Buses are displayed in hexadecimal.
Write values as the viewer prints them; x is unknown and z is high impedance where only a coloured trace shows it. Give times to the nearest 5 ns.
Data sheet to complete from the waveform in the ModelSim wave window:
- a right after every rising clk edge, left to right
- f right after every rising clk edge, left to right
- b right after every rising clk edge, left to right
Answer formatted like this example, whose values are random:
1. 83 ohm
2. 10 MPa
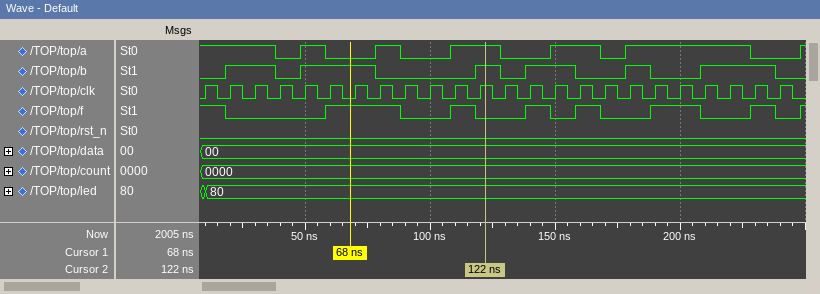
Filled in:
1. 1 1 1 0 1 0 0 1 0 0 1 1 0 0 1 1 0 1 1 1 1 1 0 0
2. 1 0 0 0 0 1 1 1 0 0 1 0 0 1 0 1 0 0 1 1 0 0 1 0
3. 0 1 1 0 1 1 1 0 0 0 0 1 0 1 1 0 0 1 0 0 1 1 1 0
